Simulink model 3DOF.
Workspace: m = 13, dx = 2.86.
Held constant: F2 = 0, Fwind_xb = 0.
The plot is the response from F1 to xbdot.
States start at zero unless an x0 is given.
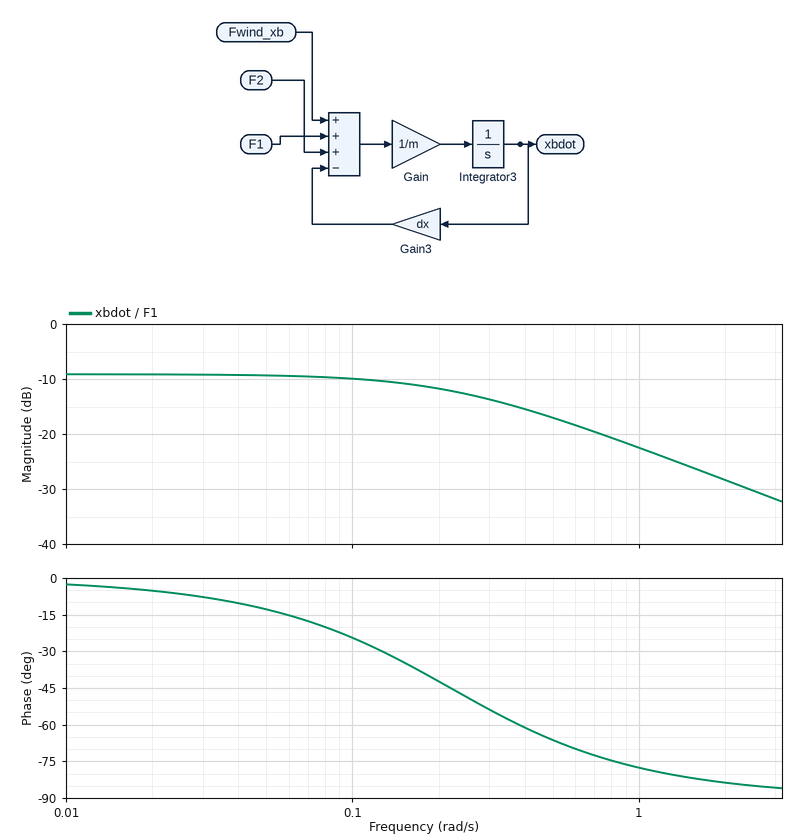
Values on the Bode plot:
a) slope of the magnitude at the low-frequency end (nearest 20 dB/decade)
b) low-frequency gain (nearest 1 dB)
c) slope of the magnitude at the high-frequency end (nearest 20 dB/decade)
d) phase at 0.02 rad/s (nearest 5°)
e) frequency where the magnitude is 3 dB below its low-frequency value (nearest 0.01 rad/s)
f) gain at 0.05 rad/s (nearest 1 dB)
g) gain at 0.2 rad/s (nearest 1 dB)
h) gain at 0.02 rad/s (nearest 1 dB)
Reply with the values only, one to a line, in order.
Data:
0 dB/decade
-9 dB
-20 dB/decade
-5°
0.22 rad/s
-9 dB
-12 dB
-9 dB
